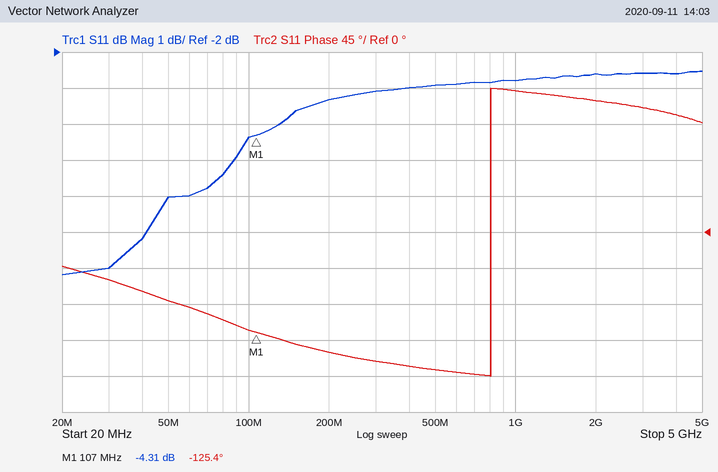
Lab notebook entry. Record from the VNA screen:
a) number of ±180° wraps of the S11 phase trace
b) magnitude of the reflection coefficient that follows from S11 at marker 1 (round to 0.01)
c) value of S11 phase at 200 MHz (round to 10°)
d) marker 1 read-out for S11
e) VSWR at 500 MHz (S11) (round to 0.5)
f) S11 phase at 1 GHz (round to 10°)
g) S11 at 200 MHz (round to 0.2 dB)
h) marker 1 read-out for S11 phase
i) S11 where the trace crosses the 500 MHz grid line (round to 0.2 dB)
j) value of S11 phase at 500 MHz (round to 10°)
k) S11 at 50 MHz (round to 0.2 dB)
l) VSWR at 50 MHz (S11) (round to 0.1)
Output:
1
0.61
-150°
-4.31 dB
6.0
180°
-3.4 dB
-125.4°
-3.0 dB
-170°
-6.0 dB
3.0
